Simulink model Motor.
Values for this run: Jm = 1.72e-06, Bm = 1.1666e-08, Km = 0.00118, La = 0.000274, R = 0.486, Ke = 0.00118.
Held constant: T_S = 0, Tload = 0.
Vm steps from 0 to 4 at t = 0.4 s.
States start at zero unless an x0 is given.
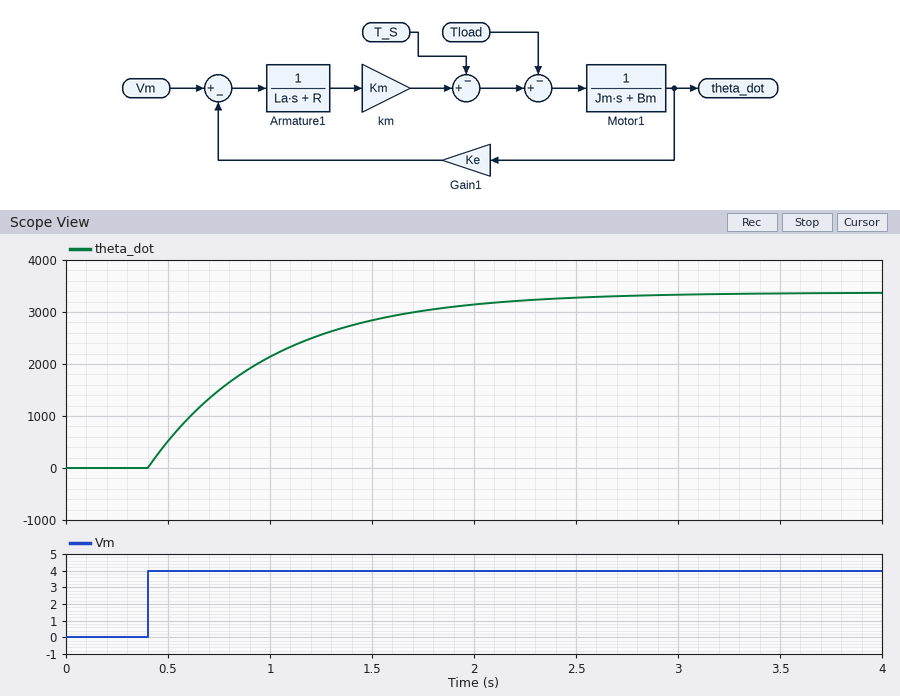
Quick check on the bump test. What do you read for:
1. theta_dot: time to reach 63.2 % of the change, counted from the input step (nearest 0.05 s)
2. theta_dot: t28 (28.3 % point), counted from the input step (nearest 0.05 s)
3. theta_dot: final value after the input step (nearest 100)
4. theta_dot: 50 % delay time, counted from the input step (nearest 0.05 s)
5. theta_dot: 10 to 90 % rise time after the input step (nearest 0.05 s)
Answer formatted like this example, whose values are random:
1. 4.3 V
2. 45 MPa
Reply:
1. 0.60 s
2. 0.20 s
3. 3400
4. 0.40 s
5. 1.30 s
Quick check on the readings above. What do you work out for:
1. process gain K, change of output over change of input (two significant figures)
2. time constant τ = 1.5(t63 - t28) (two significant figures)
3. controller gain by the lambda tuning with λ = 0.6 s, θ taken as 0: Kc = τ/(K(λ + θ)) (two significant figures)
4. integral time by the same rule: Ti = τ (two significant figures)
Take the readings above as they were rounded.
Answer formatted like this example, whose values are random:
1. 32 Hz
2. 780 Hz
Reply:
1. 850
2. 0.60 s
3. 0.0012
4. 0.60 s
